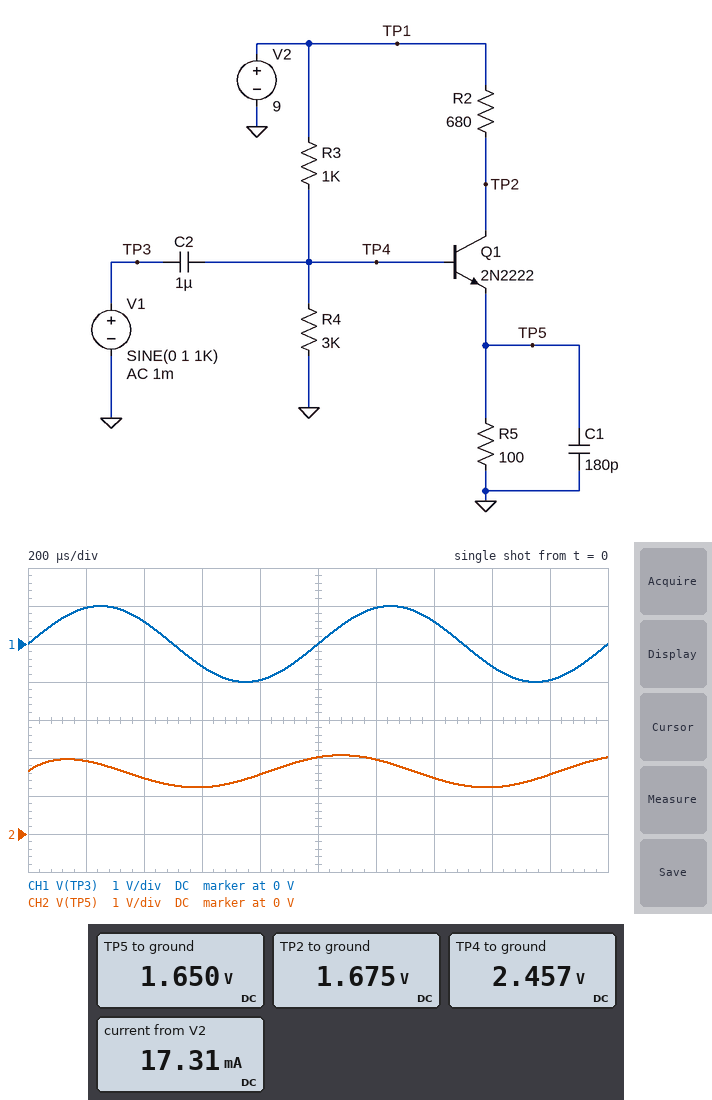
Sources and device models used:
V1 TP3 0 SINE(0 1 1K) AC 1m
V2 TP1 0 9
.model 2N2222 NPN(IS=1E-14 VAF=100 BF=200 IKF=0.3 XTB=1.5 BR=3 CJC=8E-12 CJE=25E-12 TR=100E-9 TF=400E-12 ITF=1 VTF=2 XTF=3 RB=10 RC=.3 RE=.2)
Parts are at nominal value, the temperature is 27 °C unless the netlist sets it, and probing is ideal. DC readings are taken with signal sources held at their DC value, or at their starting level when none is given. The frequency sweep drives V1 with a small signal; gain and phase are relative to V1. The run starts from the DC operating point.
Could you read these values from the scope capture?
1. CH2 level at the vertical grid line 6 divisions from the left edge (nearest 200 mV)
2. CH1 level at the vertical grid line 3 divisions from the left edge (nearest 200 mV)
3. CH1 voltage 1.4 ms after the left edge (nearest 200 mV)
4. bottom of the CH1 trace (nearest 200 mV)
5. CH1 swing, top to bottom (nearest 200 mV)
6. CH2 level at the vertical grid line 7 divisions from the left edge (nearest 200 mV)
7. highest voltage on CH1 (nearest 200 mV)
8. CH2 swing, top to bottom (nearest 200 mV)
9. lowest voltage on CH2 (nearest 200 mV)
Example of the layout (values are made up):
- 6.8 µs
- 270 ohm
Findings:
- 2.0 V
- -600 mV
- 600 mV
- -1.0 V
- 2.0 V
- 1.4 V
- 1.0 V
- 800 mV
- 1.2 V
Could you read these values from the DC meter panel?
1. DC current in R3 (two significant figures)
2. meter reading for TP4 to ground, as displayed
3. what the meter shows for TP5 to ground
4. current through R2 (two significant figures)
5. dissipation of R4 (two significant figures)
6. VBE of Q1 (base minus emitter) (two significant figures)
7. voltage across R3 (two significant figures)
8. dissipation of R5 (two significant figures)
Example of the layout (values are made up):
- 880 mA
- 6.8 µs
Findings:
- 6.5 mA
- 2.457 V
- 1.650 V
- 11 mA
- 2.0 mW
- 810 mV
- 6.5 V
- 27 mW
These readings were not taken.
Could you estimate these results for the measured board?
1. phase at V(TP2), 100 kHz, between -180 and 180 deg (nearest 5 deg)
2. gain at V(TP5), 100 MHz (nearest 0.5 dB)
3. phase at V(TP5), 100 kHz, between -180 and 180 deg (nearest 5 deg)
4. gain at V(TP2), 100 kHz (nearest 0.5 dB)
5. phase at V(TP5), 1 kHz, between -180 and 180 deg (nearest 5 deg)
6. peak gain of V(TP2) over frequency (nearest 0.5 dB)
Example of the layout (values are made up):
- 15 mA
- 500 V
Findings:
- 0 deg
- -4.5 dB
- 0 deg
- -1.5 dB
- 60 deg
- -1.0 dB
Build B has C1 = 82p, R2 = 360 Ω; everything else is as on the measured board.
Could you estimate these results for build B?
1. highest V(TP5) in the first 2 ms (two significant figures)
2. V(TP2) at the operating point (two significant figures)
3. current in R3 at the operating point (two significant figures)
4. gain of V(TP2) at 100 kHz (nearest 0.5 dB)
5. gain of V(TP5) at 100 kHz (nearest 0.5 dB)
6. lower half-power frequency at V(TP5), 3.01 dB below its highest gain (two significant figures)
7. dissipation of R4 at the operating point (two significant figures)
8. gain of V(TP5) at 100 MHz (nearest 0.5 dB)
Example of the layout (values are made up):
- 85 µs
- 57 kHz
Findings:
- 2.7 V
- 2.4 V
- 5.9 mA
- -1.5 dB
- -1.5 dB
- 2.0 kHz
- 3.3 mW
- -2.0 dB
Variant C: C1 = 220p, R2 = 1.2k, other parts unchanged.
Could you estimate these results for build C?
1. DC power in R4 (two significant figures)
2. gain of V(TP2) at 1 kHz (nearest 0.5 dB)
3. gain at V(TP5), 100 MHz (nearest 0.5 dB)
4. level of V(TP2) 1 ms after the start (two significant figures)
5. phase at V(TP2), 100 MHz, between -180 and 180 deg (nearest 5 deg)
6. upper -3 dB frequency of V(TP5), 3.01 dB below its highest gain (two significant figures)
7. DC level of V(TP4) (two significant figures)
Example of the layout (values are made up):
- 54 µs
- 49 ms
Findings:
- 1.4 mW
- -7.0 dB
- -5.5 dB
- 1.7 V
- -45 deg
- 72 MHz
- 2.1 V
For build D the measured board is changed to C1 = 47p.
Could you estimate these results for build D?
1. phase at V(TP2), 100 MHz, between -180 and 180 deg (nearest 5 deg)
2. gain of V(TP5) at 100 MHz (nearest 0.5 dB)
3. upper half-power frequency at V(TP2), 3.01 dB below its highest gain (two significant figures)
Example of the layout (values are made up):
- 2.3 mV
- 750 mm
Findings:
- -15 deg
- -1.5 dB
- 380 MHz
